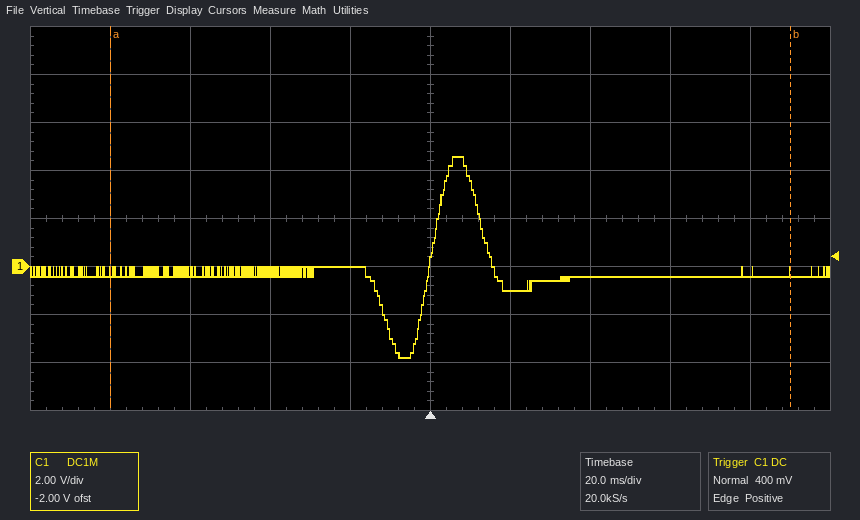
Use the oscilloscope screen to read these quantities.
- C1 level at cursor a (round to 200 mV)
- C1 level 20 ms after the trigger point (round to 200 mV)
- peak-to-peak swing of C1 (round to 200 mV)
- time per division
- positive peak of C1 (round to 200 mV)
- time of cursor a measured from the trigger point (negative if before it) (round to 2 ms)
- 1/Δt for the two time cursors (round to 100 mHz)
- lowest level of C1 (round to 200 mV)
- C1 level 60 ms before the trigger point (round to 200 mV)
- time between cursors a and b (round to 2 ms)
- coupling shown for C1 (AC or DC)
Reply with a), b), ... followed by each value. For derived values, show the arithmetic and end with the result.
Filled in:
a) -200 mV
b) -1.0 V
c) 4.6 V − (-3.8 V) = 8.4 V
d) 20 ms
e) 4.6 V
f) -80 ms
g) 1 / 170 ms ≈ 5.9 Hz
h) -3.8 V
i) -200 mV
j) 170 ms
k) DC
